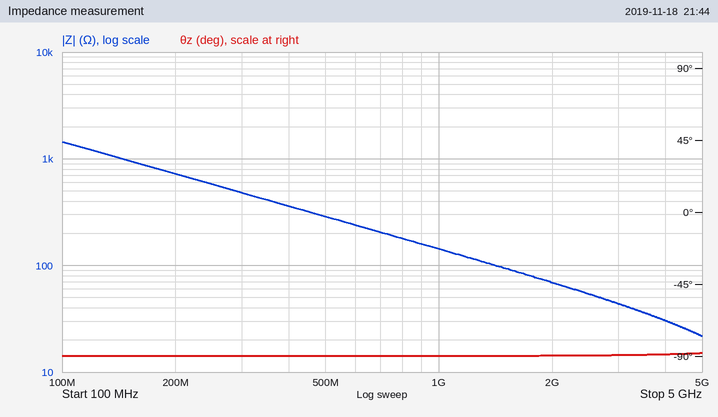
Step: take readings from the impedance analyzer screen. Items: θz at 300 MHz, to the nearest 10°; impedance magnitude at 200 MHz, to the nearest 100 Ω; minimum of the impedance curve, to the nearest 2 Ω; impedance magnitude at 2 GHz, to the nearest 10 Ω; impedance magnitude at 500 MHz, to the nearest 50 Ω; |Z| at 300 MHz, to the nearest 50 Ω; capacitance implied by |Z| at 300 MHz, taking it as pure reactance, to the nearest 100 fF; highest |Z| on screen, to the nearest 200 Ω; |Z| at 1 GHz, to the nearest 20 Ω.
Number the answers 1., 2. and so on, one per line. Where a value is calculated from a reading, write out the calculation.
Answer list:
1. -90°
2. 700 Ω
3. 22 Ω
4. 70 Ω
5. 300 Ω
6. 500 Ω
7. C = 1/(2π × 300 MHz × 500 Ω) ≈ 1.1 pF
8. 1.4 kΩ
9. 140 Ω
